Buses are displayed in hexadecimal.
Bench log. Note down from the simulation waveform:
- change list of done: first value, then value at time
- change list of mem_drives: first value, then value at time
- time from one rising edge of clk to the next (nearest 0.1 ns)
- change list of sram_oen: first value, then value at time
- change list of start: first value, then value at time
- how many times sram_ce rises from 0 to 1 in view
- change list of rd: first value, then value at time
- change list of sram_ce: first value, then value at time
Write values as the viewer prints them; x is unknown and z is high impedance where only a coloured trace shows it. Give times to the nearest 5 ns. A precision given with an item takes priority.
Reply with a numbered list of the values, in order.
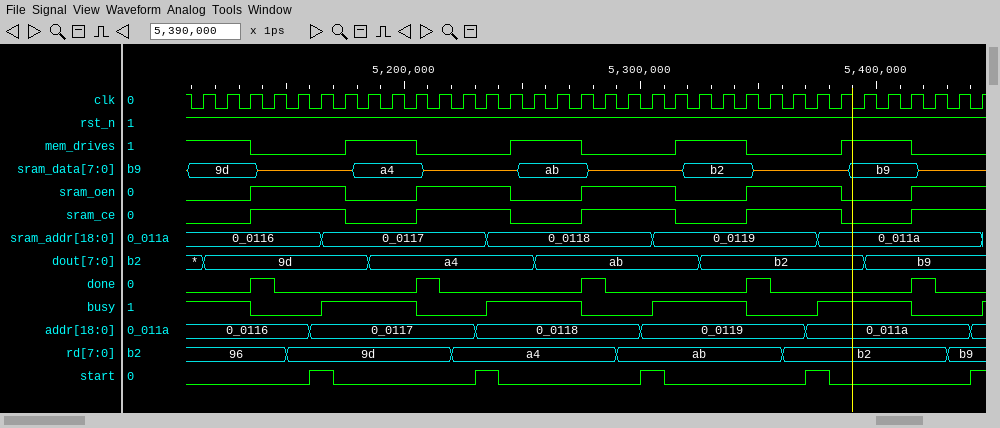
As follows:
1. 0, 1 at 5135 ns, 0 at 5145 ns, 1 at 5205 ns, 0 at 5215 ns, 1 at 5275 ns, 0 at 5285 ns, 1 at 5345 ns, 0 at 5355 ns, 1 at 5415 ns, 0 at 5425 ns
2. 1, 0 at 5135 ns, 1 at 5175 ns, 0 at 5205 ns, 1 at 5245 ns, 0 at 5275 ns, 1 at 5315 ns, 0 at 5345 ns, 1 at 5385 ns, 0 at 5415 ns
3. 10 ns
4. 0, 1 at 5135 ns, 0 at 5175 ns, 1 at 5205 ns, 0 at 5245 ns, 1 at 5275 ns, 0 at 5315 ns, 1 at 5345 ns, 0 at 5385 ns, 1 at 5415 ns
5. 0, 1 at 5160 ns, 0 at 5170 ns, 1 at 5230 ns, 0 at 5240 ns, 1 at 5300 ns, 0 at 5310 ns, 1 at 5370 ns, 0 at 5380 ns, 1 at 5440 ns
6. 5
7. 96, 9d at 5150 ns, a4 at 5220 ns, ab at 5290 ns, b2 at 5360 ns, b9 at 5430 ns
8. 0, 1 at 5135 ns, 0 at 5175 ns, 1 at 5205 ns, 0 at 5245 ns, 1 at 5275 ns, 0 at 5315 ns, 1 at 5345 ns, 0 at 5385 ns, 1 at 5415 ns
